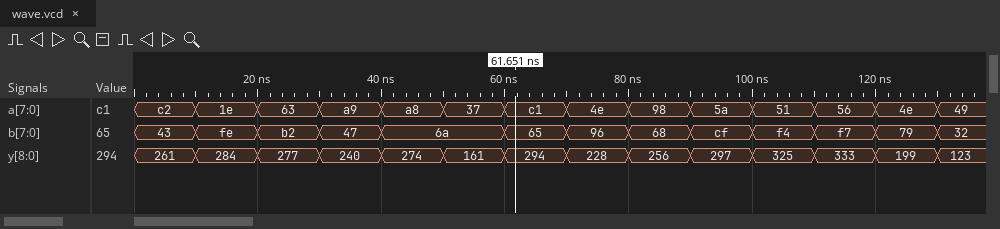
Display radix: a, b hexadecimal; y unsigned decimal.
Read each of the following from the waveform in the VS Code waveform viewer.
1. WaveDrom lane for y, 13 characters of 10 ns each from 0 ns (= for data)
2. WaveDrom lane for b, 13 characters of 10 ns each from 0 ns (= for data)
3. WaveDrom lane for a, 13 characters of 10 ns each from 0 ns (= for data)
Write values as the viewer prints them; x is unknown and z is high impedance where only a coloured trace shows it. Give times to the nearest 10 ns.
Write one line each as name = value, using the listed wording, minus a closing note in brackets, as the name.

WaveDrom lane for y, 13 characters of 10 ns each from 0 ns = {name: 'y', wave: '=============', data: '261 284 277 240 274 161 294 228 256 297 325 333 199'}
WaveDrom lane for b, 13 characters of 10 ns each from 0 ns = {name: 'b', wave: '=====.=======', data: '43 fe b2 47 6a 65 96 68 cf f4 f7 79'}
WaveDrom lane for a, 13 characters of 10 ns each from 0 ns = {name: 'a', wave: '=============', data: 'c2 1e 63 a9 a8 37 c1 4e 98 5a 51 56 4e'}
